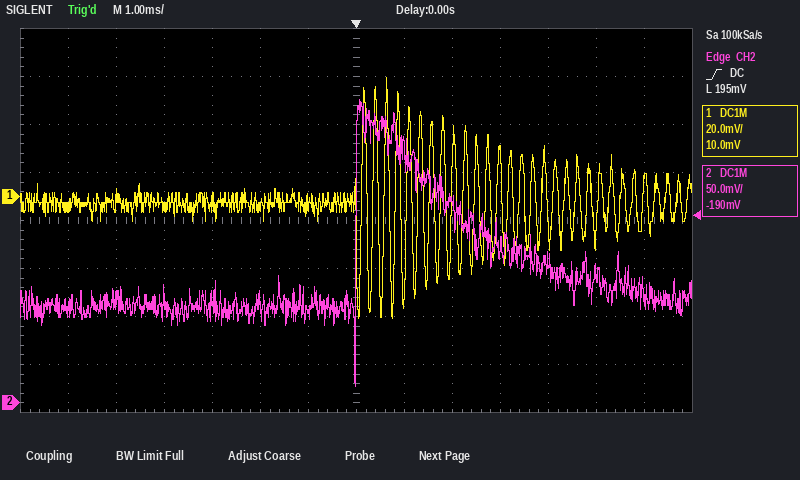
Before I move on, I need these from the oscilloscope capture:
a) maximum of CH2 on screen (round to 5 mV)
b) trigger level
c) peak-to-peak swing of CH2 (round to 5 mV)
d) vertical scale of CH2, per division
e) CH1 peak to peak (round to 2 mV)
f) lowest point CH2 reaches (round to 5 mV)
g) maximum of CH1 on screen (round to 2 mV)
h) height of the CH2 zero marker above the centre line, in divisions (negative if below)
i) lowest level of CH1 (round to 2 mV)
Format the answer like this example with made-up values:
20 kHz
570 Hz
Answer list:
315 mV
195 mV
300 mV
50 mV
100 mV
15 mV
50 mV
-3.8 div
-50 mV
